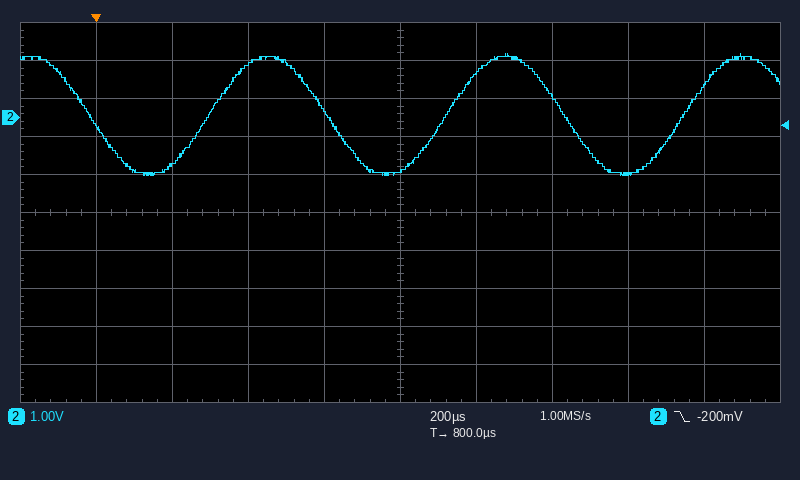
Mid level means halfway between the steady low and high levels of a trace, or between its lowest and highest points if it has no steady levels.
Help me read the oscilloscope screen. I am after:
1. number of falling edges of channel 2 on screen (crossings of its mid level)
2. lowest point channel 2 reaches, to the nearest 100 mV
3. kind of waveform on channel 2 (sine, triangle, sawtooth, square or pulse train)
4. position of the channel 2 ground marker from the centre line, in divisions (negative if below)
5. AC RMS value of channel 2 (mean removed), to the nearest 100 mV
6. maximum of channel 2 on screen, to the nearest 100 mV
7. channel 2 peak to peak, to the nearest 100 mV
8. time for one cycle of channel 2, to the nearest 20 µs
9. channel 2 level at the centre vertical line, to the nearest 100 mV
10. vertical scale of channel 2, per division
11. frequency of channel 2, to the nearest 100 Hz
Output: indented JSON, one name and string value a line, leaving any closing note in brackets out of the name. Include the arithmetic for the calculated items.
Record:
{
  "number of falling edges of channel 2 on screen": "3",
  "lowest point channel 2 reaches, to the nearest 100 mV": "-1.5 V",
  "kind of waveform on channel 2": "sine",
  "position of the channel 2 ground marker from the centre line, in divisions": "+2.5 div",
  "AC RMS value of channel 2 (mean removed), to the nearest 100 mV": "3.2 V / (2√2) ≈ 1.1 V",
  "maximum of channel 2 on screen, to the nearest 100 mV": "1.7 V",
  "channel 2 peak to peak, to the nearest 100 mV": "1.7 V − (-1.5 V) = 3.2 V",
  "time for one cycle of channel 2, to the nearest 20 µs": "620 µs",
  "channel 2 level at the centre vertical line, to the nearest 100 mV": "-1.4 V",
  "vertical scale of channel 2, per division": "1 V",
  "frequency of channel 2, to the nearest 100 Hz": "1 / 620 µs ≈ 1.6 kHz"
}
